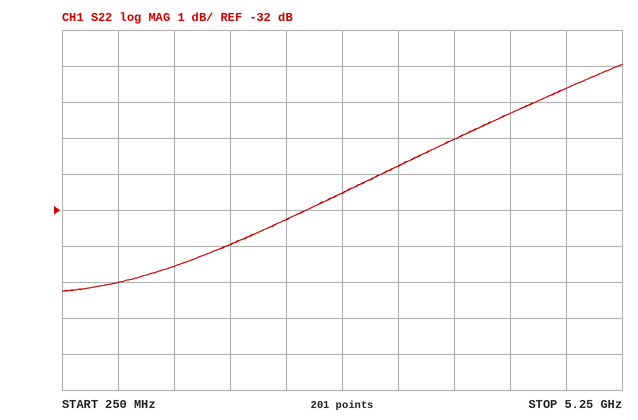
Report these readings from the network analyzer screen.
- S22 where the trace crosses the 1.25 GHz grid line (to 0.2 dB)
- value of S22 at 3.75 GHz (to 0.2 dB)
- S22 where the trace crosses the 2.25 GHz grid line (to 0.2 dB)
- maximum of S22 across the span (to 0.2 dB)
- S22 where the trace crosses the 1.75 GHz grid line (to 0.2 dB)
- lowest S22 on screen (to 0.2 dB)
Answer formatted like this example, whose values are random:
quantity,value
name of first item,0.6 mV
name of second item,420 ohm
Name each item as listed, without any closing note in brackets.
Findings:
quantity,value
S22 where the trace crosses the 1.25 GHz grid line,-33.6 dB
value of S22 at 3.75 GHz,-30.0 dB
S22 where the trace crosses the 2.25 GHz grid line,-32.2 dB
maximum of S22 across the span,-28.0 dB
S22 where the trace crosses the 1.75 GHz grid line,-33.0 dB
lowest S22 on screen,-34.2 dB
